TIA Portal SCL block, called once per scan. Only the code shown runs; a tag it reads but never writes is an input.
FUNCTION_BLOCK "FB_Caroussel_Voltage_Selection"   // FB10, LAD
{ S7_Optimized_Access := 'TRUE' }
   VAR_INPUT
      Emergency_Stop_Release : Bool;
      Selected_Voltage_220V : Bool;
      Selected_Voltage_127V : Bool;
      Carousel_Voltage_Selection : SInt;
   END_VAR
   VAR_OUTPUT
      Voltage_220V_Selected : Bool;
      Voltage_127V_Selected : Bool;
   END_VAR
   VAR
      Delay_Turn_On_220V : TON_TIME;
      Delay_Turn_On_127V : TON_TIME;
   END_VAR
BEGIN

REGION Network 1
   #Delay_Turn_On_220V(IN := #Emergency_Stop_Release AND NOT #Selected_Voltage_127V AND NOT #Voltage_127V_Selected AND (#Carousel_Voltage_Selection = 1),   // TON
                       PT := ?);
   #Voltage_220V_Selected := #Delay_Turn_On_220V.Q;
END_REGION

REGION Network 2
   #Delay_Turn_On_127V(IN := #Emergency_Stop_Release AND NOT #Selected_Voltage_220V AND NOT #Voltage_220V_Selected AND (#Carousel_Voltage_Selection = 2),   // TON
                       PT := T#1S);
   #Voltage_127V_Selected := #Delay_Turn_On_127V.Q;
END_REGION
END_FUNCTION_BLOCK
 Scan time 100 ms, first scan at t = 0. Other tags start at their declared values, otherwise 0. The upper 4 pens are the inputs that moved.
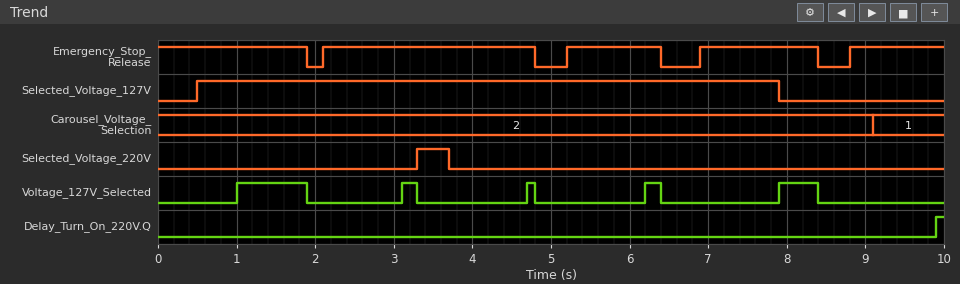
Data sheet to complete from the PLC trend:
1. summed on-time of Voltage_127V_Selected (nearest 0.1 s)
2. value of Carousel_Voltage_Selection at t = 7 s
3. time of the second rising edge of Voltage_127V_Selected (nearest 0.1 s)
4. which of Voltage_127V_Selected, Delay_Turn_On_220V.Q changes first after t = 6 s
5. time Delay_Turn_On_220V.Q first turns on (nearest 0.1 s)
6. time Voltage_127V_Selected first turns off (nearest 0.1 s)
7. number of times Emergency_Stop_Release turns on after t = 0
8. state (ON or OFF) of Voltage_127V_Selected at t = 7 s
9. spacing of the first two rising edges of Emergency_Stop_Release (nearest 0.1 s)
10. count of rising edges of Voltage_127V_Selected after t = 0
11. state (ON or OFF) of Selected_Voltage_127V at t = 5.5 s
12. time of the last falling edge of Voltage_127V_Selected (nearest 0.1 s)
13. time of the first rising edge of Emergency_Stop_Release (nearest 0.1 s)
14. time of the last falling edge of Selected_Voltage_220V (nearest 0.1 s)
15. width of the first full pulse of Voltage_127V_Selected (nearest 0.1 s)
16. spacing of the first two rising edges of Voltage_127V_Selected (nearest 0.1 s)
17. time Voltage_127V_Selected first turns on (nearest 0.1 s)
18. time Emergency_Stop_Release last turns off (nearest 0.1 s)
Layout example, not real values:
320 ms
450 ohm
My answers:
1.9 s
2
3.1 s
Voltage_127V_Selected
9.9 s
1.9 s
4
OFF
3.1 s
5
ON
8.4 s
2.1 s
3.7 s
0.9 s
2.1 s
1.0 s
8.4 s
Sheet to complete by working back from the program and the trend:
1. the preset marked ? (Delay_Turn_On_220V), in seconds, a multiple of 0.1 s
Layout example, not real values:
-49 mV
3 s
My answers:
0.8 s
